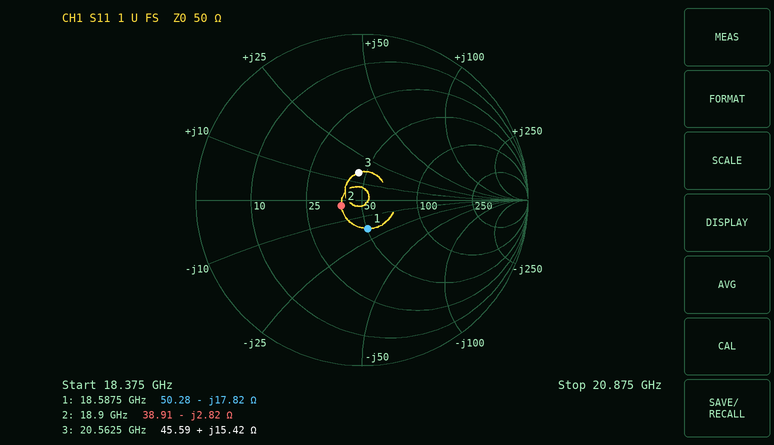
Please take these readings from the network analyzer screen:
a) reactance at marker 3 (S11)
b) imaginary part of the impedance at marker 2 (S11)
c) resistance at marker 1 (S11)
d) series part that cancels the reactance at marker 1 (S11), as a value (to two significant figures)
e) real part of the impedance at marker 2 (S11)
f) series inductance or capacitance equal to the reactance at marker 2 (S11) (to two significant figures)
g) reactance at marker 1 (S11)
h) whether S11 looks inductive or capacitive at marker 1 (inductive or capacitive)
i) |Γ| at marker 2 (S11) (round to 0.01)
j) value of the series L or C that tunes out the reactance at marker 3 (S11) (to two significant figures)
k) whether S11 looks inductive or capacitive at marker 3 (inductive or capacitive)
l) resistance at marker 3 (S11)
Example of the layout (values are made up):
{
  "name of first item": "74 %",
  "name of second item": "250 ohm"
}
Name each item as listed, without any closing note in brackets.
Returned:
{
  "reactance at marker 3": "+15.42 Ω",
  "imaginary part of the impedance at marker 2": "-2.82 Ω",
  "resistance at marker 1": "50.28 Ω",
  "series part that cancels the reactance at marker 1 (S11), as a value": "150 pH",
  "real part of the impedance at marker 2": "38.91 Ω",
  "series inductance or capacitance equal to the reactance at marker 2 (S11)": "3.0 pF",
  "reactance at marker 1": "-17.82 Ω",
  "whether S11 looks inductive or capacitive at marker 1": "capacitive",
  "|Γ| at marker 2 (S11)": "0.13",
  "value of the series L or C that tunes out the reactance at marker 3 (S11)": "500 fF",
  "whether S11 looks inductive or capacitive at marker 3": "inductive",
  "resistance at marker 3": "45.59 Ω"
}
